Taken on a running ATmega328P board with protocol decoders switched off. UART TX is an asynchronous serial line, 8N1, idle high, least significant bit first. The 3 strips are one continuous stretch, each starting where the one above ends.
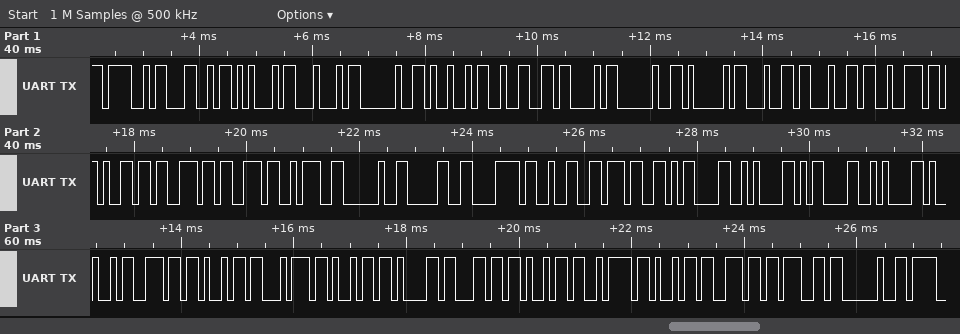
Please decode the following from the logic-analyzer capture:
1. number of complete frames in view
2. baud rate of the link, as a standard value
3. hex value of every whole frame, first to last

39
9600 baud
0x4F 0x4C 0x45 0x44 0x20 0x49 0x32 0x43 0x20 0x41 0x64 0x64 0x72 0x65 0x73 0x73 0x3A 0x20 0x30 0x78 0x32 0x37 0x0D 0x0A 0x0D 0x0A 0x49 0x6E 0x69 0x74 0x69 0x61 0x6C 0x69 0x7A 0x69 0x6E 0x67 0x20
